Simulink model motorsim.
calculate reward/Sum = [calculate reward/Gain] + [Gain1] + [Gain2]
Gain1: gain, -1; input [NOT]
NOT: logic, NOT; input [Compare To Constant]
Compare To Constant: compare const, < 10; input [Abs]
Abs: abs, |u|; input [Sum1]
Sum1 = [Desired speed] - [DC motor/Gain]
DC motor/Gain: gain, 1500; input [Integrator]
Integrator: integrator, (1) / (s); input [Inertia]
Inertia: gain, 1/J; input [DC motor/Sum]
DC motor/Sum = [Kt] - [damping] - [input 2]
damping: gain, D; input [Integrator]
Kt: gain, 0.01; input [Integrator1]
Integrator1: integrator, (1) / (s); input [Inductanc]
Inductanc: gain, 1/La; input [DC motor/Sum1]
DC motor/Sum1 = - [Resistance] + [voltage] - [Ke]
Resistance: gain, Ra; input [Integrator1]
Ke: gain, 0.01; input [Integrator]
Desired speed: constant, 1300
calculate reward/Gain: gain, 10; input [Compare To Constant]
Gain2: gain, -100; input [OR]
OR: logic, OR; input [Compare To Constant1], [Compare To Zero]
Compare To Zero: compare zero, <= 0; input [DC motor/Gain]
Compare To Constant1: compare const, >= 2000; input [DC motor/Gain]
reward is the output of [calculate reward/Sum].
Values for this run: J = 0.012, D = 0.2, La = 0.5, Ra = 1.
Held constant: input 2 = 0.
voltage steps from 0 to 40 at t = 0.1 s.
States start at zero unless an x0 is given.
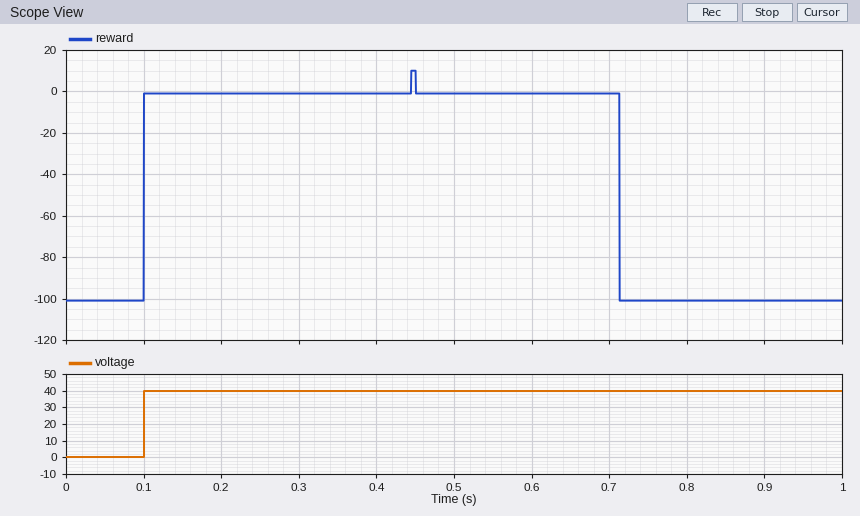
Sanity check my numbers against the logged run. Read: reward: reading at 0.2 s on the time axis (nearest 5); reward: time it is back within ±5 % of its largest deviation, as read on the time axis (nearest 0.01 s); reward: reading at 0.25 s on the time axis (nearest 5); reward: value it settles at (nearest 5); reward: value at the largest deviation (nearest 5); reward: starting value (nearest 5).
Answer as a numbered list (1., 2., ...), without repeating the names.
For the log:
1. 0
2. 0.71 s
3. 0
4. -100
5. 10
6. -100
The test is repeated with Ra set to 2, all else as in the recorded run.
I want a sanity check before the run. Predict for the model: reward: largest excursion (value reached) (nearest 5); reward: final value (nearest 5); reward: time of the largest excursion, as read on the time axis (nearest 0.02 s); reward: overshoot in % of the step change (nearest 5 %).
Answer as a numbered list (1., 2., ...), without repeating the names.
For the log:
1. 10
2. 0
3. 0.66 s
4. 10 %
